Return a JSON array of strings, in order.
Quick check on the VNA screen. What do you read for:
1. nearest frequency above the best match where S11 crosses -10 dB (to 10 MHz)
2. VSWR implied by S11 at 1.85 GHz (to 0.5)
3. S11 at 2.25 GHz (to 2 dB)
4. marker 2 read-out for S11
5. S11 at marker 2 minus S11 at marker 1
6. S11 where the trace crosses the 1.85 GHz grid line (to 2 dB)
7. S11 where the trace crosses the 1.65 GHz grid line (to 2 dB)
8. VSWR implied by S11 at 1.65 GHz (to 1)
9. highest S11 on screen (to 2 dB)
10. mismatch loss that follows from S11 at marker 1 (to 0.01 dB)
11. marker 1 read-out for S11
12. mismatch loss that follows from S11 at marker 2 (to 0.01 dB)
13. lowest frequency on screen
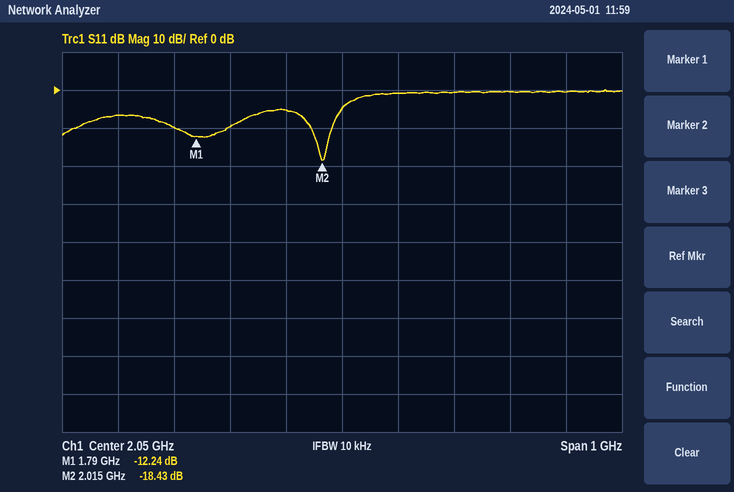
["2.03 GHz", "2.0", "0 dB", "-18.43 dB", "-6.19 dB", "-10 dB", "-6 dB", "3", "0 dB", "0.27 dB", "-12.24 dB", "0.06 dB", "1.55 GHz"]
